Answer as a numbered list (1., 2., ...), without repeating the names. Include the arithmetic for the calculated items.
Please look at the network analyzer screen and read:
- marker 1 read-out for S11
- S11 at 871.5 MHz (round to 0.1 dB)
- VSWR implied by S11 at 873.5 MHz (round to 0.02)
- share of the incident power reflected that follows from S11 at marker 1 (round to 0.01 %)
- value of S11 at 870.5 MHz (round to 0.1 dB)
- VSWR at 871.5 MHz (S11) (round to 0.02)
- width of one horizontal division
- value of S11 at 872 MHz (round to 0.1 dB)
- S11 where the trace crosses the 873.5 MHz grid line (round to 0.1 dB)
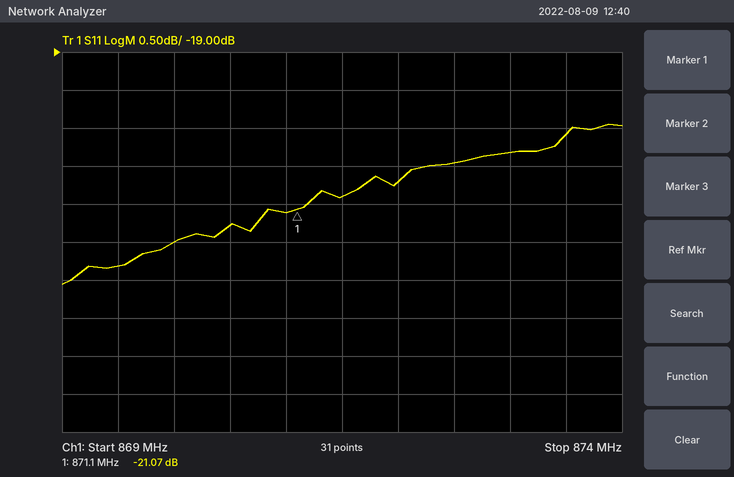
1. -21.07 dB
2. -20.9 dB
3. |Γ| = 10^(-20.1/20) = 0.0989; VSWR = (1 + 0.0989)/(1 − 0.0989) ≈ 1.22
4. 10^(-21.07/10) ≈ 0.78 %
5. -21.3 dB
6. |Γ| = 10^(-20.9/20) = 0.0902; VSWR = (1 + 0.0902)/(1 − 0.0902) ≈ 1.20
7. 500 kHz
8. -20.7 dB
9. -20.1 dB
